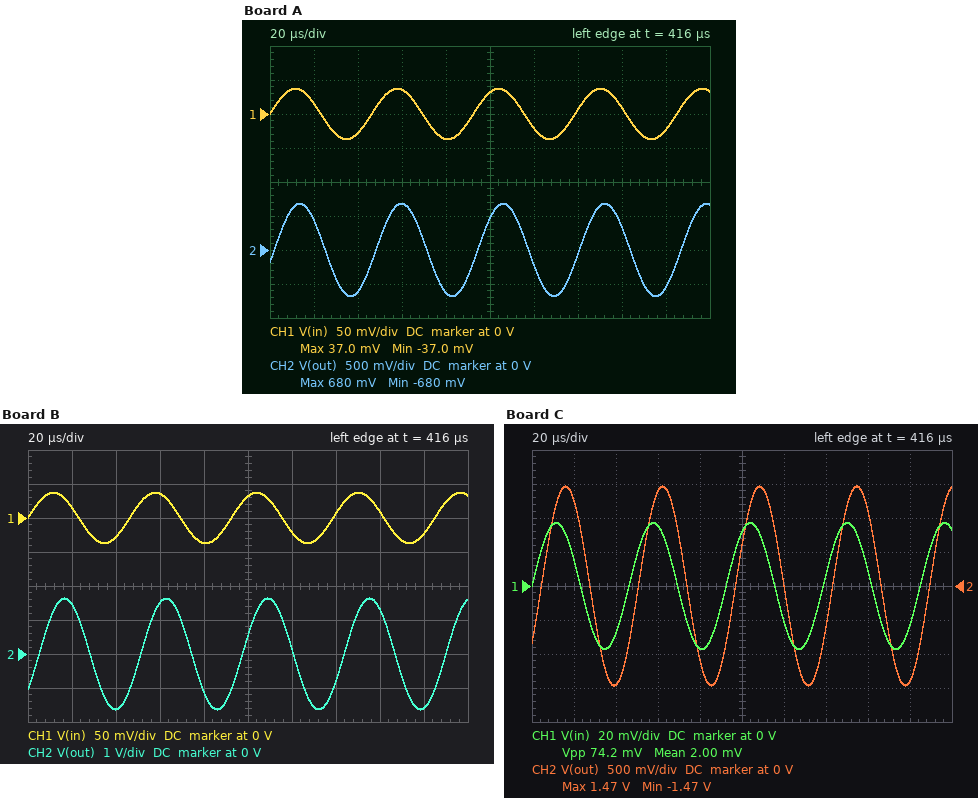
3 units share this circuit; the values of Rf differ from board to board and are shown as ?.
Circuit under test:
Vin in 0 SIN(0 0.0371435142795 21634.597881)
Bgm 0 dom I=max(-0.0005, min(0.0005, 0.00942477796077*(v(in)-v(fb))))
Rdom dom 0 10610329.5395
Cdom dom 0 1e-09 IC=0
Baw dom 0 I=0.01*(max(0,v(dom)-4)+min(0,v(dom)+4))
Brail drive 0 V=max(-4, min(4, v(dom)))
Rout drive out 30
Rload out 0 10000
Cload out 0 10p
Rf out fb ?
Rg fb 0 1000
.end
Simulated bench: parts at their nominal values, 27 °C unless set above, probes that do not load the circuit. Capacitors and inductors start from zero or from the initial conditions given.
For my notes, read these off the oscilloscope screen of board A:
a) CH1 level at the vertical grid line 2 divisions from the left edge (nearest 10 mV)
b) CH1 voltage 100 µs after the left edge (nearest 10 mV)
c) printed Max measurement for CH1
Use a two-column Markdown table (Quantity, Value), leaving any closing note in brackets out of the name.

| Quantity | Value |
|---|---|
| CH1 level at the vertical grid line 2 divisions from the left edge | -30 mV |
| CH1 voltage 100 µs after the left edge | 30 mV |
| printed Max measurement for CH1 | 37.0 mV |
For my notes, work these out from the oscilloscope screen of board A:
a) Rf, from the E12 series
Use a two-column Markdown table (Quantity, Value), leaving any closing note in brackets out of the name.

| Quantity | Value |
|---|---|
| Rf, from the E12 series | 18 kΩ |
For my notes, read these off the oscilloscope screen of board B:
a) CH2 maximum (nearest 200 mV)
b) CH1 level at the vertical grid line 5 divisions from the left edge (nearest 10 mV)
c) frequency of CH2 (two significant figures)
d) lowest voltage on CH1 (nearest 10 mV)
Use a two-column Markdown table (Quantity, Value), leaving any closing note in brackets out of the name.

| Quantity | Value |
|---|---|
| CH2 maximum | 1.6 V |
| CH1 level at the vertical grid line 5 divisions from the left edge | 30 mV |
| frequency of CH2 | 22 kHz |
| lowest voltage on CH1 | -40 mV |
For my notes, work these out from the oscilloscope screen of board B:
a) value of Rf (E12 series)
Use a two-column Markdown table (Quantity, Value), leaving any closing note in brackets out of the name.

| Quantity | Value |
|---|---|
| value of Rf | 56 kΩ |
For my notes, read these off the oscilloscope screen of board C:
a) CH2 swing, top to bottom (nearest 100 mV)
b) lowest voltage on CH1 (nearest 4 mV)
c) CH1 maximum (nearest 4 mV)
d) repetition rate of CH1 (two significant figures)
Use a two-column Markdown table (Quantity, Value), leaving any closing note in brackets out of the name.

| Quantity | Value |
|---|---|
| CH2 swing, top to bottom | 2.9 V |
| lowest voltage on CH1 | -36 mV |
| CH1 maximum | 36 mV |
| repetition rate of CH1 | 22 kHz |
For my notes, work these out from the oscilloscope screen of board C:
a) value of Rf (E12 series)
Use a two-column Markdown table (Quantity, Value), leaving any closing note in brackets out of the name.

| Quantity | Value |
|---|---|
| value of Rf | 47 kΩ |
